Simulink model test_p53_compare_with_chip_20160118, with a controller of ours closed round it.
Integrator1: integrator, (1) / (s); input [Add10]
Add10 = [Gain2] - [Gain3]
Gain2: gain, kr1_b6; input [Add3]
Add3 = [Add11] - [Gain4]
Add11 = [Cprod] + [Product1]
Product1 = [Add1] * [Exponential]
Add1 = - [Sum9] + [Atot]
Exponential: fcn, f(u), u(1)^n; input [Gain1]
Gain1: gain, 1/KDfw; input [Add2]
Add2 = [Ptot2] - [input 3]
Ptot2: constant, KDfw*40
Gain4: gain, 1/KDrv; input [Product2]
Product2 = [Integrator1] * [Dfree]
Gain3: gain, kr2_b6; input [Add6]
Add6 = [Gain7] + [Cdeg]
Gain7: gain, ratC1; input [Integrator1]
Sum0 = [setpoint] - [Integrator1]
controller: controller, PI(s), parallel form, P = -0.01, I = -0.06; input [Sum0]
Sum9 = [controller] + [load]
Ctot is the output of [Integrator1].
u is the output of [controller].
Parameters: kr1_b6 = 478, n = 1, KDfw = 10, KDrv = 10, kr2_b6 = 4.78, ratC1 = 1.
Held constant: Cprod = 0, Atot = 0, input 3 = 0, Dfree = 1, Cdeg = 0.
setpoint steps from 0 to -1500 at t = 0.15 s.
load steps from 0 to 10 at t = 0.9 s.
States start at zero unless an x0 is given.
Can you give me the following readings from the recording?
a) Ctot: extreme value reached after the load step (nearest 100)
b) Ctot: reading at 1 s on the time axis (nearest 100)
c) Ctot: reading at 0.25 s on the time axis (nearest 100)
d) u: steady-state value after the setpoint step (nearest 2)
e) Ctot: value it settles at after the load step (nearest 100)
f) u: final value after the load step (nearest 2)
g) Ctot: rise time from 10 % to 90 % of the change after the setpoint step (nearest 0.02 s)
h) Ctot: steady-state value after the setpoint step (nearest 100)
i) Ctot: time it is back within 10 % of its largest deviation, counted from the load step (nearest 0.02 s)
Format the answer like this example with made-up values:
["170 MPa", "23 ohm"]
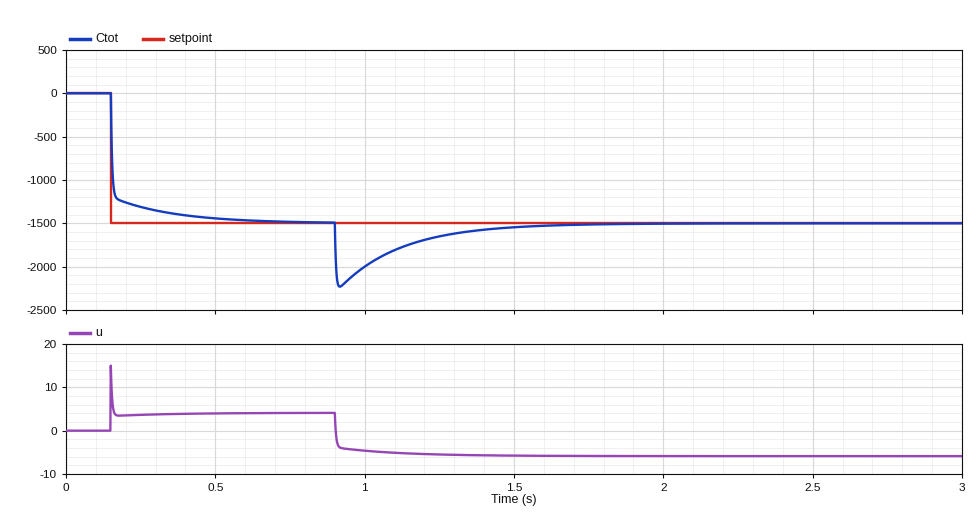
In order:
["-2200", "-2000", "-1300", "4", "-1500", "-6", "0.14 s", "-1500", "0.50 s"]
